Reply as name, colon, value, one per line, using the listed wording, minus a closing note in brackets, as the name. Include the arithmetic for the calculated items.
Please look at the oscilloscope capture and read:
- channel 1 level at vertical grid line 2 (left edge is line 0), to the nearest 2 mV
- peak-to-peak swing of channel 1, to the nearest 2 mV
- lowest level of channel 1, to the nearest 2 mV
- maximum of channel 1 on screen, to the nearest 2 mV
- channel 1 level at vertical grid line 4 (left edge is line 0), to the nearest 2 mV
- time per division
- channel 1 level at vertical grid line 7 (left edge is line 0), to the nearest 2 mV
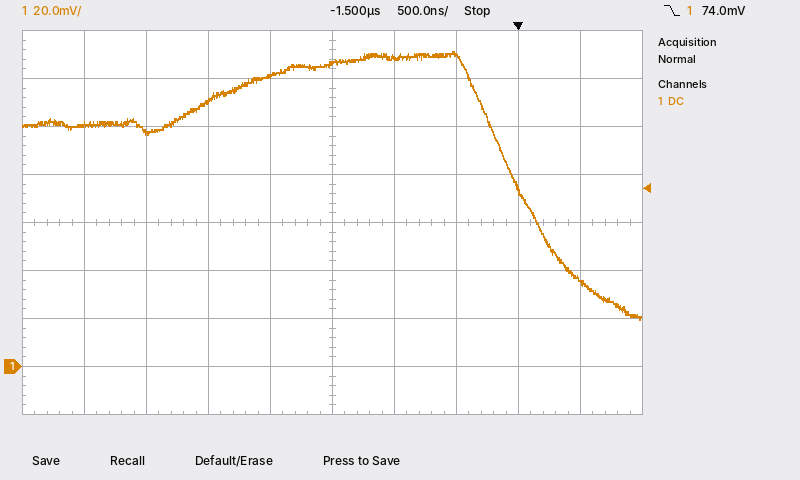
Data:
channel 1 level at vertical grid line 2 (left edge is line 0), to the nearest 2 mV: 98 mV
peak-to-peak swing of channel 1, to the nearest 2 mV: 132 mV − (20 mV) = 112 mV
lowest level of channel 1, to the nearest 2 mV: 20 mV
maximum of channel 1 on screen, to the nearest 2 mV: 132 mV
channel 1 level at vertical grid line 4 (left edge is line 0), to the nearest 2 mV: 122 mV
time per division: 500 ns
channel 1 level at vertical grid line 7 (left edge is line 0), to the nearest 2 mV: 130 mV
